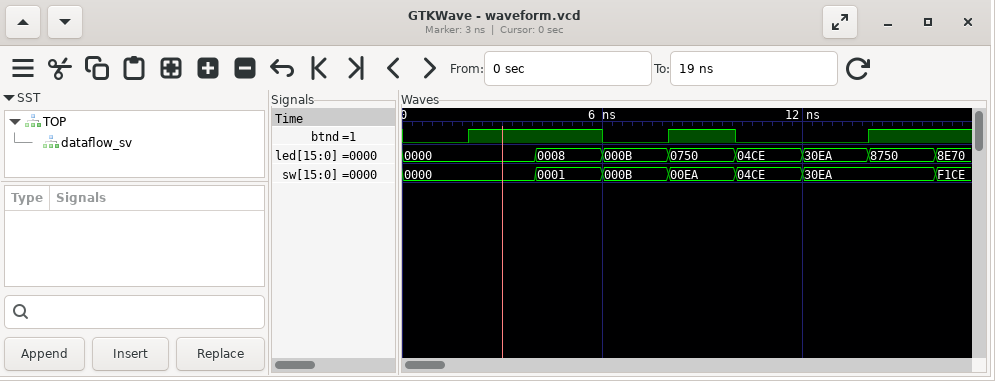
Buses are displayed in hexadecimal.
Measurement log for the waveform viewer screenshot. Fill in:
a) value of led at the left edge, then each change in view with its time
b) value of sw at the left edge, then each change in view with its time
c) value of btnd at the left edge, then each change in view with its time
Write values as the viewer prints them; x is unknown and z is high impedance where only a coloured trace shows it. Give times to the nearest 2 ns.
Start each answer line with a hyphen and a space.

- 0000, 0008 at 4 ns, 000B at 6 ns, 0750 at 8 ns, 04CE at 10 ns, 30EA at 12 ns, 8750 at 14 ns, 8E70 at 16 ns
- 0000, 0001 at 4 ns, 000B at 6 ns, 00EA at 8 ns, 04CE at 10 ns, 30EA at 12 ns, F1CE at 16 ns
- 0, 1 at 2 ns, 0 at 6 ns, 1 at 8 ns, 0 at 10 ns, 1 at 14 ns
